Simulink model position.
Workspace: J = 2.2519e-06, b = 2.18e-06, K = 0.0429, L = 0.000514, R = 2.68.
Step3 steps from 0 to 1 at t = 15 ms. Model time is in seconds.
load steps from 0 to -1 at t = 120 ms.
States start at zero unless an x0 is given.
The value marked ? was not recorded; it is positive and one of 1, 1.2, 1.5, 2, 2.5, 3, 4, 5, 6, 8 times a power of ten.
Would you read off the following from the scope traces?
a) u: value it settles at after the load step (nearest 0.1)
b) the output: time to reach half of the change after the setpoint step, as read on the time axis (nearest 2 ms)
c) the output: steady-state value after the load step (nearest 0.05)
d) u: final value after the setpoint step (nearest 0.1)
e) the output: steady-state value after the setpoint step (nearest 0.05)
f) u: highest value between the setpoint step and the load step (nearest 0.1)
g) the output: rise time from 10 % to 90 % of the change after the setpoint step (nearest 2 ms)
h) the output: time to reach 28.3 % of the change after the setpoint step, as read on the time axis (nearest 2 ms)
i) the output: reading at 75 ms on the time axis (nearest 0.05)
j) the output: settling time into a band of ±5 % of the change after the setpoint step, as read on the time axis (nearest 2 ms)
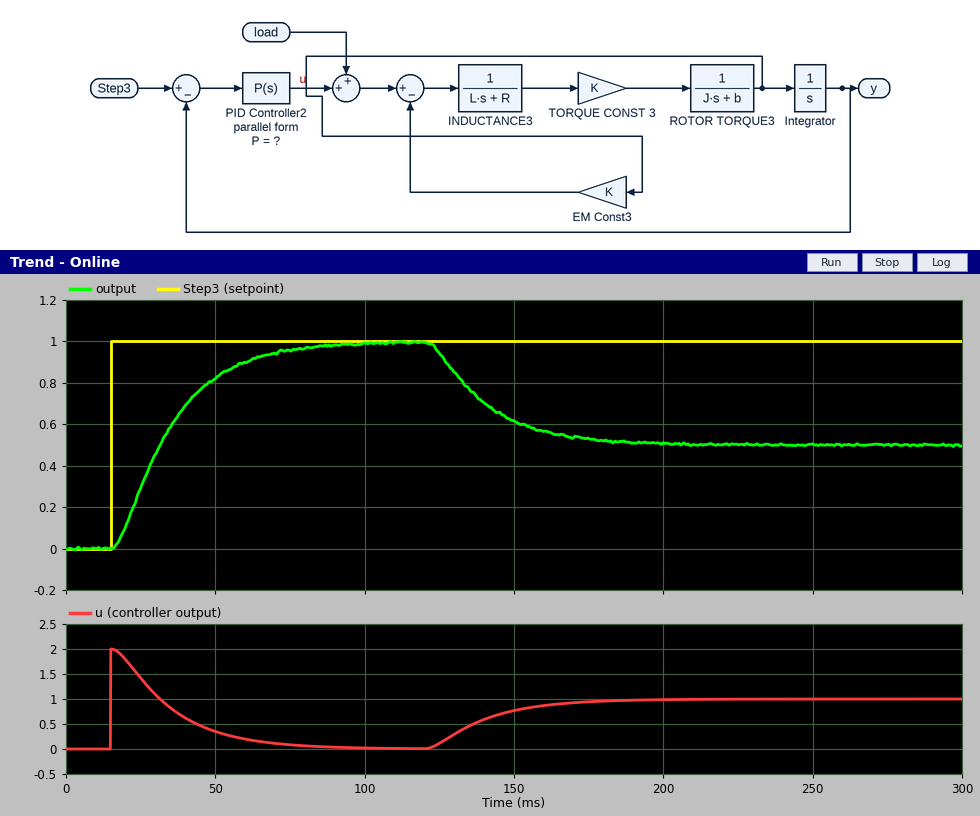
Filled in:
1.0
32 ms
0.50
0.0
1.00
2.0
40 ms
24 ms
0.95
72 ms
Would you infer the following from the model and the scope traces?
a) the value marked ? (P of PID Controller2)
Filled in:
2
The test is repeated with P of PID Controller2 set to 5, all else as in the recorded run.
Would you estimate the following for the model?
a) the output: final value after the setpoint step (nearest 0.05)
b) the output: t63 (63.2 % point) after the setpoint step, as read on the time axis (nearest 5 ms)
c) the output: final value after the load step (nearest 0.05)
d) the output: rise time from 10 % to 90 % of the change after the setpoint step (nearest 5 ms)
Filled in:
1.00
25 ms
0.80
15 ms
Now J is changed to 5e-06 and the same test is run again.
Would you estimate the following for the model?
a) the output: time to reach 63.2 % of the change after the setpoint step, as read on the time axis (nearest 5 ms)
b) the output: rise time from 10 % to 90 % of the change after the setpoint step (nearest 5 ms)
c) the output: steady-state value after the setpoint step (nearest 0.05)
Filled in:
40 ms
35 ms
1.00
